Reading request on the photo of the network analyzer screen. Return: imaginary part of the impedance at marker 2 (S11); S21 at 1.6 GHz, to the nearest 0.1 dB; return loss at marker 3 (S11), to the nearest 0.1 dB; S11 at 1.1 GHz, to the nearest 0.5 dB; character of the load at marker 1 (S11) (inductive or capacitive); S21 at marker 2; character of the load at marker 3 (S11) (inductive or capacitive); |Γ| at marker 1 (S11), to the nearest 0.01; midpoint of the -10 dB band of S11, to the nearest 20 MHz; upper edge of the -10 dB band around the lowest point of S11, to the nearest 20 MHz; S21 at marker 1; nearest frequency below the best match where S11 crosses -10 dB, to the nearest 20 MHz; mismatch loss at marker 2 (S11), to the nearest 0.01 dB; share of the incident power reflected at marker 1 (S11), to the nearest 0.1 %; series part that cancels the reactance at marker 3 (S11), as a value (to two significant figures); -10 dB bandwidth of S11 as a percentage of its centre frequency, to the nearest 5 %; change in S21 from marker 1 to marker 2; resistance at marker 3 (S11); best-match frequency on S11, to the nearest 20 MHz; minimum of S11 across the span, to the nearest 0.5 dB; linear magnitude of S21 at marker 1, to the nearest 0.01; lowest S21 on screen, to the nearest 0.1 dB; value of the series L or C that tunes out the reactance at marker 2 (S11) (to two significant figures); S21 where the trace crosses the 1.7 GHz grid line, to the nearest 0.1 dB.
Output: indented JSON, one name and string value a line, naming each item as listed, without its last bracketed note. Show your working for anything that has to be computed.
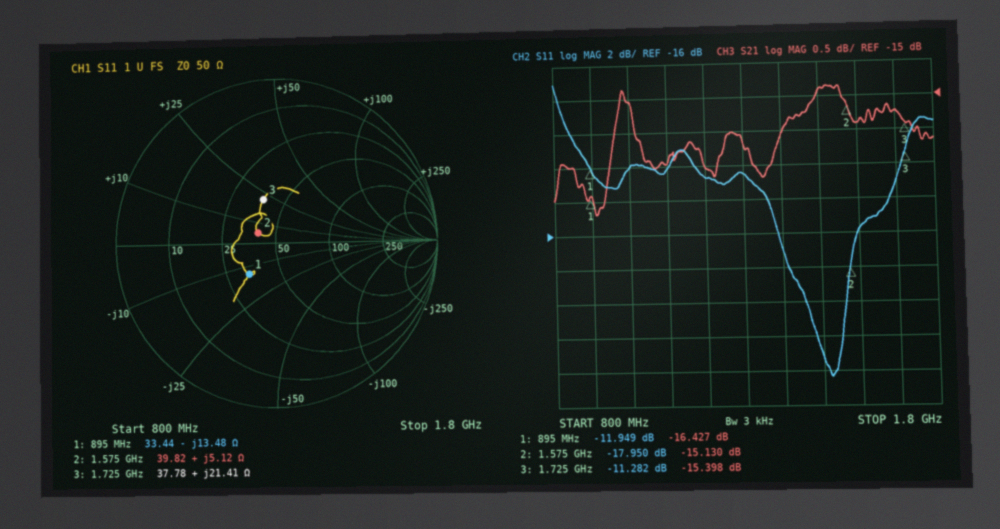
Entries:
{
  "imaginary part of the impedance at marker 2": "+5.12 Ω",
  "S21 at 1.6 GHz, to the nearest 0.1 dB": "-15.4 dB",
  "return loss at marker 3 (S11), to the nearest 0.1 dB": "11.3 dB",
  "S11 at 1.1 GHz, to the nearest 0.5 dB": "-12.0 dB",
  "character of the load at marker 1 (S11)": "capacitive",
  "S21 at marker 2": "-15.130 dB",
  "character of the load at marker 3 (S11)": "inductive",
  "|Γ| at marker 1 (S11), to the nearest 0.01": "0.25",
  "midpoint of the -10 dB band of S11, to the nearest 20 MHz": "1.30 GHz",
  "upper edge of the -10 dB band around the lowest point of S11, to the nearest 20 MHz": "1.74 GHz",
  "S21 at marker 1": "-16.427 dB",
  "nearest frequency below the best match where S11 crosses -10 dB, to the nearest 20 MHz": "840 MHz",
  "mismatch loss at marker 2 (S11), to the nearest 0.01 dB": "−10 log10(1 − 10^(-17.95/10)) ≈ 0.07 dB",
  "share of the incident power reflected at marker 1 (S11), to the nearest 0.1 %": "10^(-11.949/10) ≈ 6.4 %",
  "series part that cancels the reactance at marker 3 (S11), as a value": "C = 1/(2π × 1.725 GHz × 21.41 Ω) ≈ 4.3 pF",
  "-10 dB bandwidth of S11 as a percentage of its centre frequency, to the nearest 5 %": "900 MHz / 1.29 GHz ≈ 70 %",
  "change in S21 from marker 1 to marker 2": "-15.13 − (-16.427) = 1.297 dB",
  "resistance at marker 3": "37.78 Ω",
  "best-match frequency on S11, to the nearest 20 MHz": "1.52 GHz",
  "minimum of S11 across the span, to the nearest 0.5 dB": "-24.5 dB",
  "linear magnitude of S21 at marker 1, to the nearest 0.01": "10^(-16.427/20) ≈ 0.15",
  "lowest S21 on screen, to the nearest 0.1 dB": "-16.7 dB",
  "value of the series L or C that tunes out the reactance at marker 2 (S11)": "C = 1/(2π × 1.575 GHz × 5.12 Ω) ≈ 20 pF",
  "S21 where the trace crosses the 1.7 GHz grid line, to the nearest 0.1 dB": "-15.2 dB"
}
